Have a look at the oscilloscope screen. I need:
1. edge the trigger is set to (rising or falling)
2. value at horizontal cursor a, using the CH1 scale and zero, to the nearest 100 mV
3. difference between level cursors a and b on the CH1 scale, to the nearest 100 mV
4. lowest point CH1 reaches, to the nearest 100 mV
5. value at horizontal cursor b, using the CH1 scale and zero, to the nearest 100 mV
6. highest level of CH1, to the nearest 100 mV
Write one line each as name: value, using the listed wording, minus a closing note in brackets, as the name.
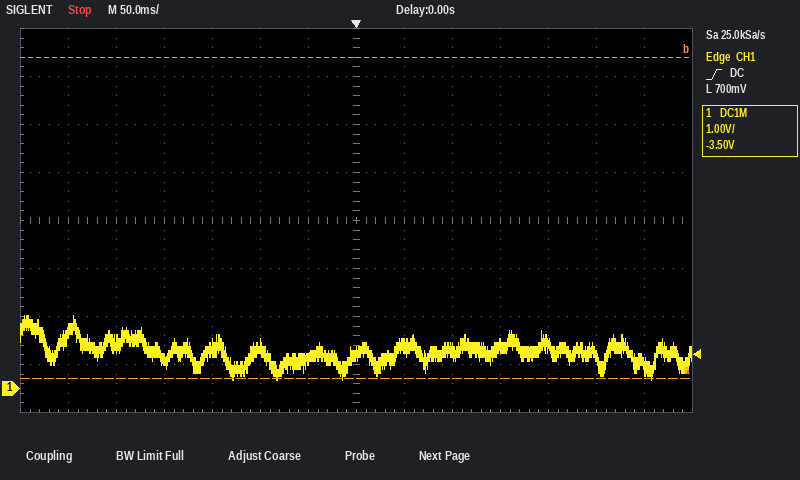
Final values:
edge the trigger is set to: rising
value at horizontal cursor a, using the CH1 scale and zero, to the nearest 100 mV: 200 mV
difference between level cursors a and b on the CH1 scale, to the nearest 100 mV: 6.7 V
lowest point CH1 reaches, to the nearest 100 mV: 200 mV
value at horizontal cursor b, using the CH1 scale and zero, to the nearest 100 mV: 6.9 V
highest level of CH1, to the nearest 100 mV: 1.5 V
